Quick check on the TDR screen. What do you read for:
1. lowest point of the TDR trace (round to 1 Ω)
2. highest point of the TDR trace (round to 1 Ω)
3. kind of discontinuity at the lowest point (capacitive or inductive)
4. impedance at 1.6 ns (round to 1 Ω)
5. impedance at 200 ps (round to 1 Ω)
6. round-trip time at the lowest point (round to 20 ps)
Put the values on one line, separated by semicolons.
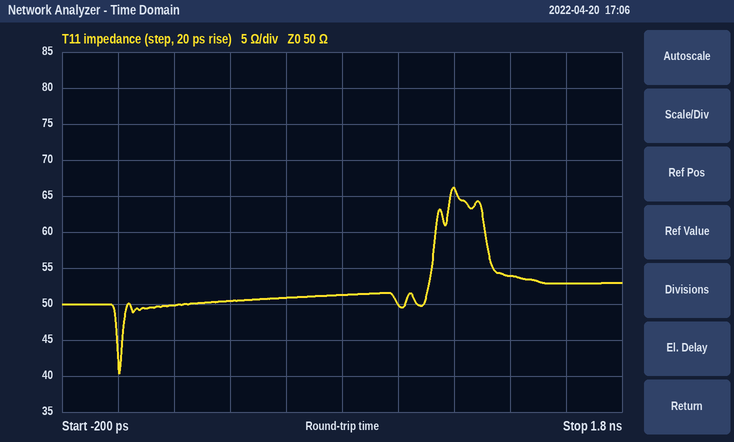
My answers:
40 Ω; 66 Ω; capacitive; 53 Ω; 50 Ω; 0 ps
